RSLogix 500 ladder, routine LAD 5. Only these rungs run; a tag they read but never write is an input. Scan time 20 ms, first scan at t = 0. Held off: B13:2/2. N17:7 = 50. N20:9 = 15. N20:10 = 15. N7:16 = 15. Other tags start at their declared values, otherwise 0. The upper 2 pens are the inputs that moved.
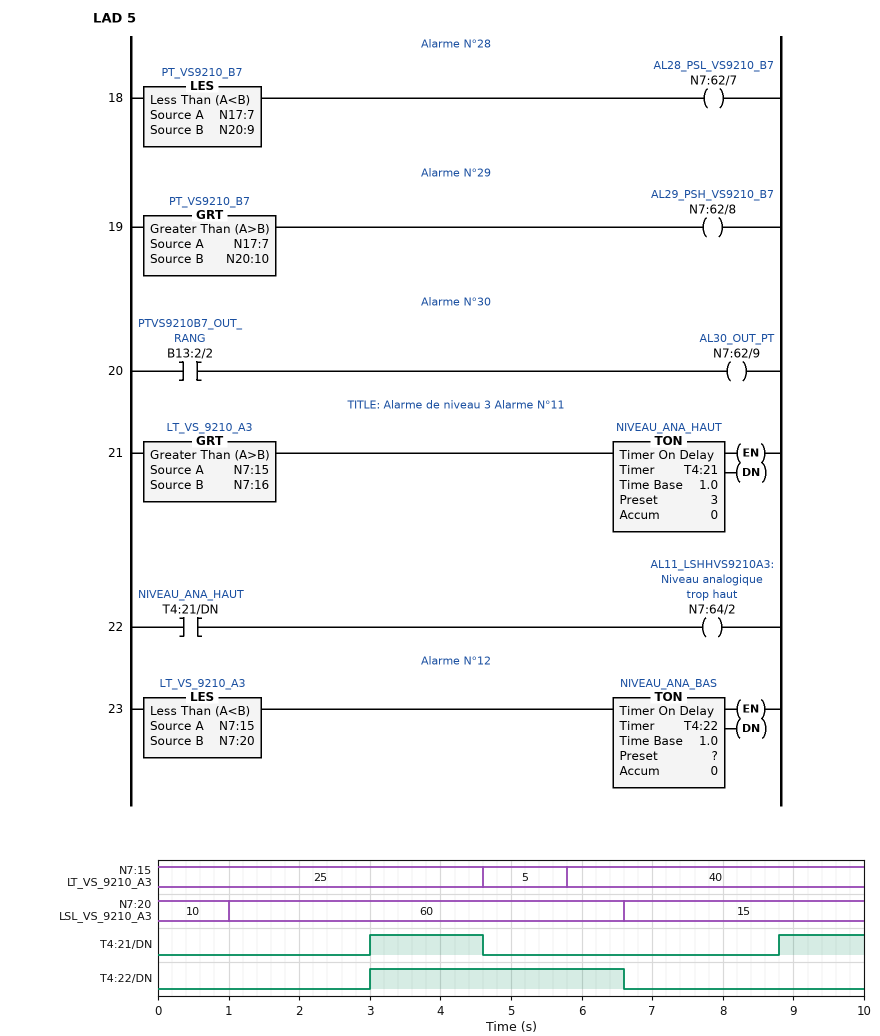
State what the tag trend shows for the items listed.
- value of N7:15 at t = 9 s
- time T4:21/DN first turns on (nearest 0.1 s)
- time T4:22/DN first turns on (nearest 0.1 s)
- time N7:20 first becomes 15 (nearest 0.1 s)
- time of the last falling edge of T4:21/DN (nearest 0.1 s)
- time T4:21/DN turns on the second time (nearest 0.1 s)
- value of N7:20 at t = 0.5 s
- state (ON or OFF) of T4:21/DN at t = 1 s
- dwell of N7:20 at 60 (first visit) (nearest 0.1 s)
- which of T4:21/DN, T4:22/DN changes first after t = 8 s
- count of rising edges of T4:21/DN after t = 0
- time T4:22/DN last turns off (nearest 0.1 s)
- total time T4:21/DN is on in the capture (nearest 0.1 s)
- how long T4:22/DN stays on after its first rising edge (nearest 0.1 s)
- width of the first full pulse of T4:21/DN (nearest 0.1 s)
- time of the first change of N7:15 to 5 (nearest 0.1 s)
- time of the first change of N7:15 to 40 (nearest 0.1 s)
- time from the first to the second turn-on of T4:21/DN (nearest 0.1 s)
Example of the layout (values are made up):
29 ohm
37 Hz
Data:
40
3.0 s
3.0 s
6.6 s
4.6 s
8.8 s
10
OFF
5.6 s
T4:21/DN
2
6.6 s
2.8 s
3.6 s
1.6 s
4.6 s
5.8 s
5.8 s
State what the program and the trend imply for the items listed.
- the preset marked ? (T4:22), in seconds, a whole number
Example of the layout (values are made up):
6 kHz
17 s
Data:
2 s
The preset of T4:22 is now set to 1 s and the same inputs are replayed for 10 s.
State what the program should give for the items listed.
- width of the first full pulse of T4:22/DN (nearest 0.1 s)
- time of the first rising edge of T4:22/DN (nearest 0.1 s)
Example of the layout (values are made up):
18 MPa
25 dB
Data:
4.6 s
2.0 s
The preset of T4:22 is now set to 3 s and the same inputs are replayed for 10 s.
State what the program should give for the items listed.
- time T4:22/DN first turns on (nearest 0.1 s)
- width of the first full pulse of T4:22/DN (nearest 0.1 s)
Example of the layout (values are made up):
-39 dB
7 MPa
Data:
4.0 s
2.6 s
